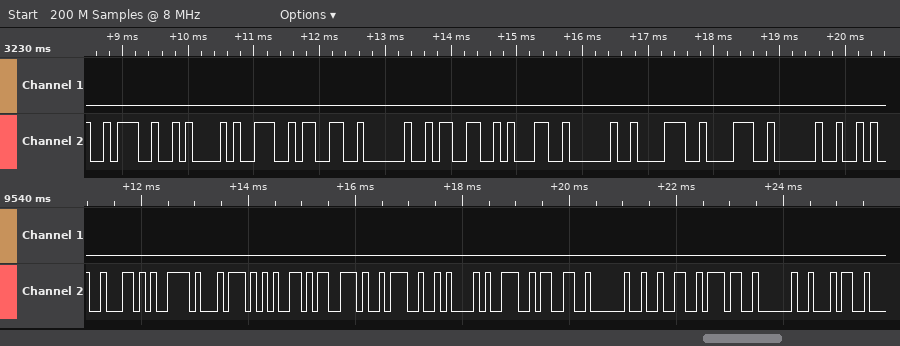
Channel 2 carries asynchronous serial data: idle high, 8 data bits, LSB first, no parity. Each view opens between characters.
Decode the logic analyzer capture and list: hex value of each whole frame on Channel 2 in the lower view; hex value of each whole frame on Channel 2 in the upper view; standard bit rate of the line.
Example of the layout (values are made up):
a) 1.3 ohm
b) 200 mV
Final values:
a) 62, 79, 74, 65, 73, 3A, 0A, 39, 33, 20, 32, 37, 20, 34
b) 3A, 0A, 39, 33, 20, 33, 31, 20, 38, 38, 20
c) 9600 baud
